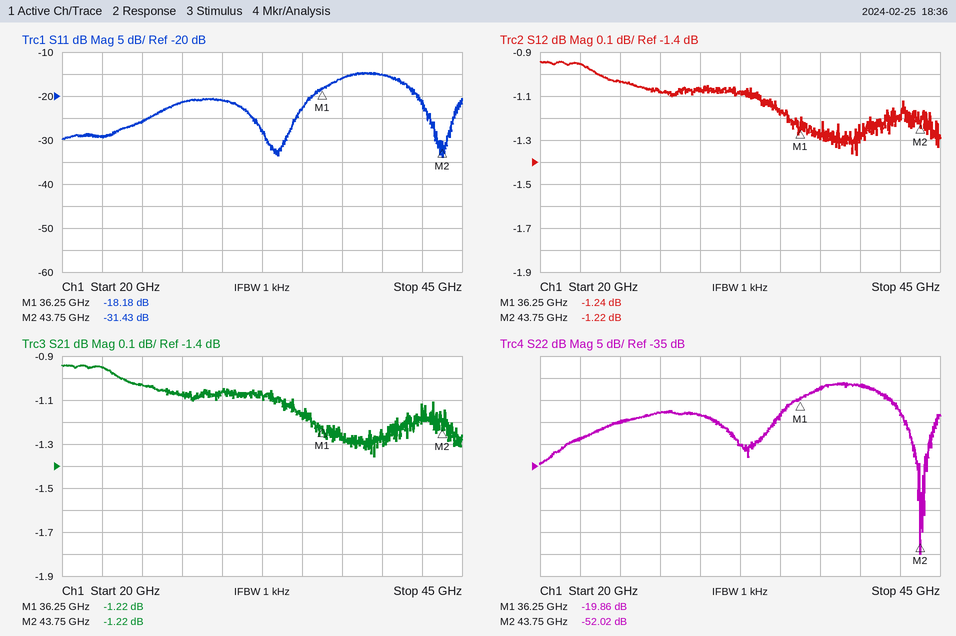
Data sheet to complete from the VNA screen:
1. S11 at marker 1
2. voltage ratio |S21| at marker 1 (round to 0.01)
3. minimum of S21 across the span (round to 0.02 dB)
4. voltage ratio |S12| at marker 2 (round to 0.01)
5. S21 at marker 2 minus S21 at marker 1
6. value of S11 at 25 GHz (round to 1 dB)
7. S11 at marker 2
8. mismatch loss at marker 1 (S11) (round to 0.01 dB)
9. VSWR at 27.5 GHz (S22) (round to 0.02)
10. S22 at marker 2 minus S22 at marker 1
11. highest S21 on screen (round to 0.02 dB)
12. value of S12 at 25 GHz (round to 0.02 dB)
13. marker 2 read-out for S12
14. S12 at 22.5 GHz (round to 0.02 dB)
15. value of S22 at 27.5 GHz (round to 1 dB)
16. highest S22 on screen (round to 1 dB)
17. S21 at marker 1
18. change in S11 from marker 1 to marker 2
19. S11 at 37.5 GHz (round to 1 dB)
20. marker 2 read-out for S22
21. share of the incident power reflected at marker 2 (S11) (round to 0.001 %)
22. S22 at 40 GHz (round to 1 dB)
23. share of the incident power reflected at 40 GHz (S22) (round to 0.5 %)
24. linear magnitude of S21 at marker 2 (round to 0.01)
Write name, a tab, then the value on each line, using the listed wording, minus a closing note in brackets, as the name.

S11 at marker 1	-18.18 dB
voltage ratio |S21| at marker 1	0.87
minimum of S21 across the span	-1.36 dB
voltage ratio |S12| at marker 2	0.87
S21 at marker 2 minus S21 at marker 1	0.00 dB
value of S11 at 25 GHz	-26 dB
S11 at marker 2	-31.43 dB
mismatch loss at marker 1 (S11)	0.07 dB
VSWR at 27.5 GHz (S22)	1.16
S22 at marker 2 minus S22 at marker 1	-32.16 dB
highest S21 on screen	-0.94 dB
value of S12 at 25 GHz	-1.04 dB
marker 2 read-out for S12	-1.22 dB
S12 at 22.5 GHz	-0.96 dB
value of S22 at 27.5 GHz	-23 dB
highest S22 on screen	-16 dB
S21 at marker 1	-1.22 dB
change in S11 from marker 1 to marker 2	-13.25 dB
S11 at 37.5 GHz	-16 dB
marker 2 read-out for S22	-52.02 dB
share of the incident power reflected at marker 2 (S11)	0.072 %
S22 at 40 GHz	-17 dB
share of the incident power reflected at 40 GHz (S22)	2.0 %
linear magnitude of S21 at marker 2	0.87
